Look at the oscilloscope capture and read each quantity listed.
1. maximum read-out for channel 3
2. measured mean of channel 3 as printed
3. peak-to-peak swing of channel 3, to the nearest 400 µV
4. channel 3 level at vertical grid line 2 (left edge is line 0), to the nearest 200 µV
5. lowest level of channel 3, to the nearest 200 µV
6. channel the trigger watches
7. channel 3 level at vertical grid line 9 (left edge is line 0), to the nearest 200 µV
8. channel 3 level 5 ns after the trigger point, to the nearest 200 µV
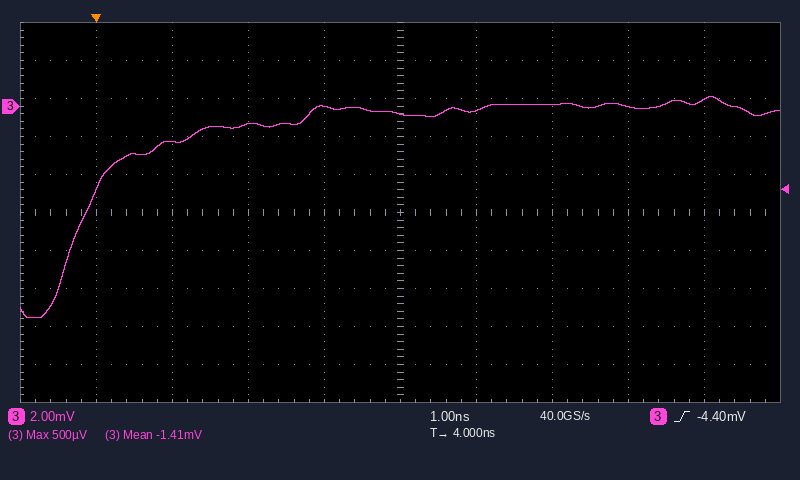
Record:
500 µV
-1.41 mV
11.6 mV
-1.8 mV
-11.2 mV
channel 3
400 µV
-200 µV
